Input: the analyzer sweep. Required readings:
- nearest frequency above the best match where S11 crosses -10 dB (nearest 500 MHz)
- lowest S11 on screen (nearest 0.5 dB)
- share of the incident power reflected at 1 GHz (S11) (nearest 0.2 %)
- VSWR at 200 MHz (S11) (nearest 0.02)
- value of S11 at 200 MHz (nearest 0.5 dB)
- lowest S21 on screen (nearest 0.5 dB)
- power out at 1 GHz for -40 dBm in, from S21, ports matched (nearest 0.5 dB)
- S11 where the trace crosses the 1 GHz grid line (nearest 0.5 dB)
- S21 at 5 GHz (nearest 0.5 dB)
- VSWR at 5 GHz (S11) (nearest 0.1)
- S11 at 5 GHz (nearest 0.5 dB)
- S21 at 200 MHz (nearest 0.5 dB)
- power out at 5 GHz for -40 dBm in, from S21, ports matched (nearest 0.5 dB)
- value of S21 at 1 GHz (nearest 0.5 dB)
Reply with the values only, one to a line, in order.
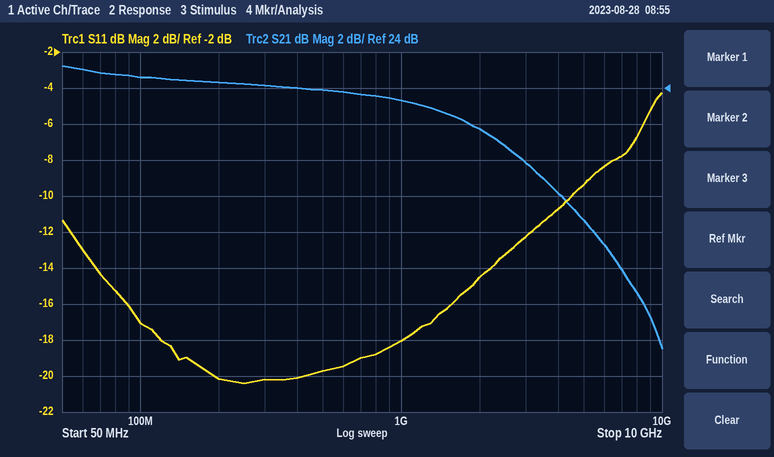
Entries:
4.5 GHz
-20.5 dB
1.6 %
1.22
-20.0 dB
9.5 dB
-16.5 dBm
-18.0 dB
16.5 dB
2.0
-9.5 dB
24.5 dB
-23.5 dBm
23.5 dB
